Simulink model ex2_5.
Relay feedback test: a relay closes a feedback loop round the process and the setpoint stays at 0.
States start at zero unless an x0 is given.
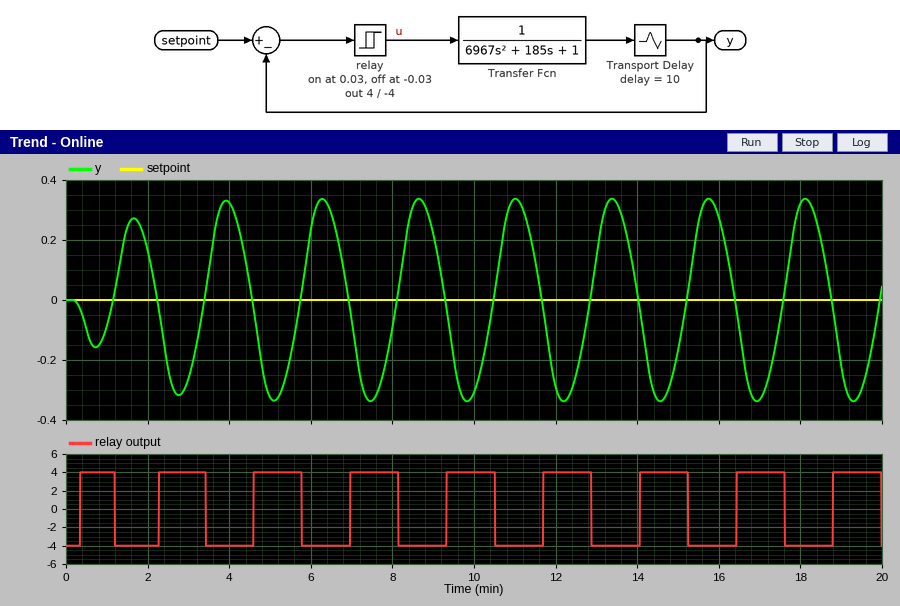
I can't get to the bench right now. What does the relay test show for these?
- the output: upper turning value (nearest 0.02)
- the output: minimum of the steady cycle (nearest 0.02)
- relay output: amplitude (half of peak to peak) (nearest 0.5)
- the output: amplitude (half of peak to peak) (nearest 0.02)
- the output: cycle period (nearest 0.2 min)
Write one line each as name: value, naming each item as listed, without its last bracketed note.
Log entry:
the output: upper turning value: 0.34
the output: minimum of the steady cycle: -0.34
relay output: amplitude (half of peak to peak): 4.0
the output: amplitude (half of peak to peak): 0.34
the output: cycle period: 2.4 min
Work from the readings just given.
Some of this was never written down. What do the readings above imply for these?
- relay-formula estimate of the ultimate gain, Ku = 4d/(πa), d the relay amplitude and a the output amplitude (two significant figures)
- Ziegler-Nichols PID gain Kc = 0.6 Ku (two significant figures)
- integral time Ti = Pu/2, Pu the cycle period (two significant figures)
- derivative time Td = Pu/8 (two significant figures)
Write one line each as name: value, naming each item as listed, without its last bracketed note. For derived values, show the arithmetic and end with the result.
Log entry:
relay-formula estimate of the ultimate gain, Ku = 4d/(πa), d the relay amplitude and a the output amplitude: 4 × 4 / (π × 0.34) = 15
Ziegler-Nichols PID gain Kc = 0.6 Ku: 0.6 × 15 = 9.0
integral time Ti = Pu/2, Pu the cycle period: 2.4 / 2 = 1.2 min
derivative time Td = Pu/8: 2.4 / 8 = 0.30 min
